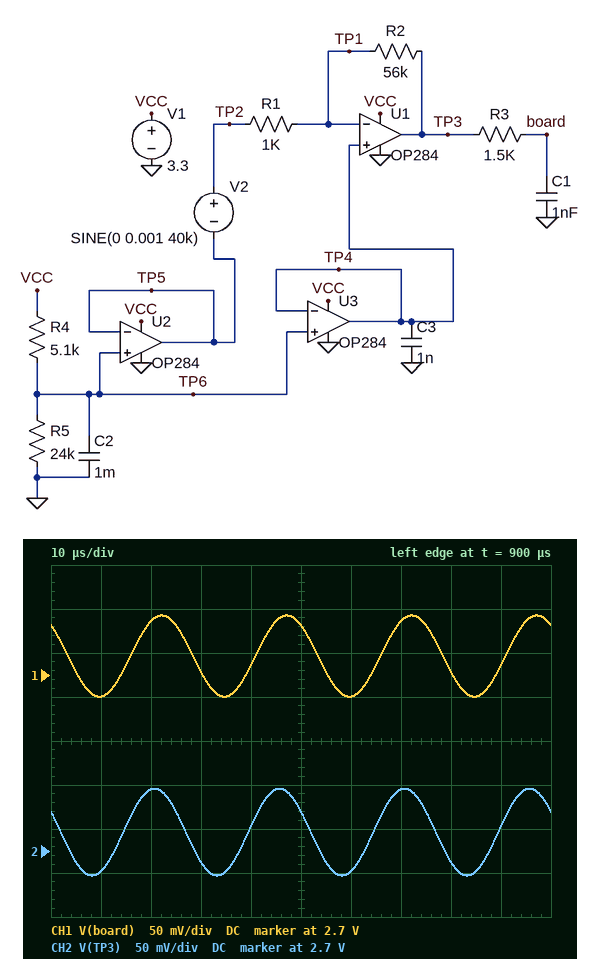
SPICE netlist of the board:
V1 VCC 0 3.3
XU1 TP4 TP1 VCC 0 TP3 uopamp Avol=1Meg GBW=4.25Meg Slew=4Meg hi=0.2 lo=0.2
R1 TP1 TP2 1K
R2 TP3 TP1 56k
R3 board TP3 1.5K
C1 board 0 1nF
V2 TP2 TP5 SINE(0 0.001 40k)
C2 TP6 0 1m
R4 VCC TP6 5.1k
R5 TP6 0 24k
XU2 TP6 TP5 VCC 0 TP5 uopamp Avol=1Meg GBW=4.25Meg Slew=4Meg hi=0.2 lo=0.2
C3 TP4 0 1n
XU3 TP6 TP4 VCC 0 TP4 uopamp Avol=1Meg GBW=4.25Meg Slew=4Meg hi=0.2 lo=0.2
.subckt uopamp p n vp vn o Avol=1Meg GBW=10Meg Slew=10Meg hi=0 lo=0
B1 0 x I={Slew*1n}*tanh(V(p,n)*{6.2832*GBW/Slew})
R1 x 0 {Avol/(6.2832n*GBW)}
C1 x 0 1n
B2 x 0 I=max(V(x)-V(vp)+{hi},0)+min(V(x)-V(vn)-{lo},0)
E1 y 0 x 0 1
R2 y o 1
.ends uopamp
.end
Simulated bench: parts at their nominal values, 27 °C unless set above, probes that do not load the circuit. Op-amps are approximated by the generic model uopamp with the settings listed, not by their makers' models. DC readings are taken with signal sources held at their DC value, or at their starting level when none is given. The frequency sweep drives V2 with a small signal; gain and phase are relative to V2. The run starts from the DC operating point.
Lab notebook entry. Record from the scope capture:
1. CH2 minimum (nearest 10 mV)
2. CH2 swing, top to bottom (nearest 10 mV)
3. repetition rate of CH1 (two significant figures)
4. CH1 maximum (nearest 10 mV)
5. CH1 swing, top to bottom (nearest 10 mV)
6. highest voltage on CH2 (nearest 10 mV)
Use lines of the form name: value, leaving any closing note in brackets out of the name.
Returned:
CH2 minimum: 2.67 V
CH2 swing, top to bottom: 100 mV
repetition rate of CH1: 40 kHz
CH1 maximum: 2.77 V
CH1 swing, top to bottom: 90 mV
highest voltage on CH2: 2.77 V
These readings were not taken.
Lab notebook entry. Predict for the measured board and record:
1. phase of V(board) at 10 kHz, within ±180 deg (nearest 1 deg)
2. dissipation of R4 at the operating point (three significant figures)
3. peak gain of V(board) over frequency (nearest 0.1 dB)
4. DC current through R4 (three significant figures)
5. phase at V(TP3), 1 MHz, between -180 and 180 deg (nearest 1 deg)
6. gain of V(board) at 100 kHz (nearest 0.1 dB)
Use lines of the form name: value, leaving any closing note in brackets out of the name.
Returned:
phase of V(board) at 10 kHz, within ±180 deg: 167 deg
dissipation of R4 at the operating point: 65.6 µW
peak gain of V(board) over frequency: 35.0 dB
DC current through R4: 113 µA
phase at V(TP3), 1 MHz, between -180 and 180 deg: 94 deg
gain of V(board) at 100 kHz: 27.7 dB
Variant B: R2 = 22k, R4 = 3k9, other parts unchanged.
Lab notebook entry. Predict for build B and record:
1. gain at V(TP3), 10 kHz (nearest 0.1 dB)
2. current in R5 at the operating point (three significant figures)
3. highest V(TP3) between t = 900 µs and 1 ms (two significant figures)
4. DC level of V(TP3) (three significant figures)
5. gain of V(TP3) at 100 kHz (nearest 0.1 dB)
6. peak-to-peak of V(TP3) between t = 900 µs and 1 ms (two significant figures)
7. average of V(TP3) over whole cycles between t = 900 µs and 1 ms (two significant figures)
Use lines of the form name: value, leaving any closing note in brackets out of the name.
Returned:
gain at V(TP3), 10 kHz: 26.8 dB
current in R5 at the operating point: 118 µA
highest V(TP3) between t = 900 µs and 1 ms: 2.9 V
DC level of V(TP3): 2.84 V
gain of V(TP3) at 100 kHz: 25.7 dB
peak-to-peak of V(TP3) between t = 900 µs and 1 ms: 43 mV
average of V(TP3) over whole cycles between t = 900 µs and 1 ms: 2.8 V
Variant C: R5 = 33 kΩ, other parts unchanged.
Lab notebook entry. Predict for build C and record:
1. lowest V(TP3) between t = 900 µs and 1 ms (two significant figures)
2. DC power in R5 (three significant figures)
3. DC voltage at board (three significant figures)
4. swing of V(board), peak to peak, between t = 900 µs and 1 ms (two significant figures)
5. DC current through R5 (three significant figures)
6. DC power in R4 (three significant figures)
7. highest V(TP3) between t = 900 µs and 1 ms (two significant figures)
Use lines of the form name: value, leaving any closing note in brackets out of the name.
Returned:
lowest V(TP3) between t = 900 µs and 1 ms: 2.8 V
DC power in R5: 248 µW
DC voltage at board: 2.86 V
swing of V(board), peak to peak, between t = 900 µs and 1 ms: 92 mV
DC current through R5: 86.6 µA
DC power in R4: 38.3 µW
highest V(TP3) between t = 900 µs and 1 ms: 2.9 V
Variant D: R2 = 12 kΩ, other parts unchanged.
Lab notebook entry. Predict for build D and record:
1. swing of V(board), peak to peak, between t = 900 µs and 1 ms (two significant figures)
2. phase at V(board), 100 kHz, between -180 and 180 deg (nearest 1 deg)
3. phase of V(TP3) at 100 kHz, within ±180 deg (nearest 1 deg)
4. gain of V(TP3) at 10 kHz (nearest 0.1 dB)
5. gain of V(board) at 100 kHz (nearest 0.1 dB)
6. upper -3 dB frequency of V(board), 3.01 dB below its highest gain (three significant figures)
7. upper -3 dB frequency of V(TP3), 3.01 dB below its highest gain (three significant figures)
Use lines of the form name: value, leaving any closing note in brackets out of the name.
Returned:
swing of V(board), peak to peak, between t = 900 µs and 1 ms: 22 mV
phase at V(board), 100 kHz, between -180 and 180 deg: 120 deg
phase of V(TP3) at 100 kHz, within ±180 deg: 163 deg
gain of V(TP3) at 10 kHz: 21.6 dB
gain of V(board) at 100 kHz: 18.4 dB
upper -3 dB frequency of V(board), 3.01 dB below its highest gain: 97.1 kHz
upper -3 dB frequency of V(TP3), 3.01 dB below its highest gain: 327 kHz
